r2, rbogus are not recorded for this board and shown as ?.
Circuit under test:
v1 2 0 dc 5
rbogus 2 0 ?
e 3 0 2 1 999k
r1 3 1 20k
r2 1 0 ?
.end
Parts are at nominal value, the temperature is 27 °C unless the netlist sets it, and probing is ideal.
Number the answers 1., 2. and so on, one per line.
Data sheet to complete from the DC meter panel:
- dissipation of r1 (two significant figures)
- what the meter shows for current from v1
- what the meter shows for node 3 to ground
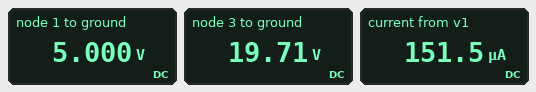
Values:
1. 11 mW
2. 151.5 µA
3. 19.71 V
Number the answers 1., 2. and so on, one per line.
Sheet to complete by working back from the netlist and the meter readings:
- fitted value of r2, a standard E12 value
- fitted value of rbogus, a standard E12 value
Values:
1. 6.8 kΩ
2. 33 kΩ
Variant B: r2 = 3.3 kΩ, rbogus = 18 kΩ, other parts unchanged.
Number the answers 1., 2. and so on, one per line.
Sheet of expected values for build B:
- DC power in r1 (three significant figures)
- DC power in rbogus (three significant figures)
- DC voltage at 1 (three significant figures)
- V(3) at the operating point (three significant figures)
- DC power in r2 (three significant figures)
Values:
1. 45.9 mW
2. 1.39 mW
3. 5.00 V
4. 35.3 V
5. 7.58 mW
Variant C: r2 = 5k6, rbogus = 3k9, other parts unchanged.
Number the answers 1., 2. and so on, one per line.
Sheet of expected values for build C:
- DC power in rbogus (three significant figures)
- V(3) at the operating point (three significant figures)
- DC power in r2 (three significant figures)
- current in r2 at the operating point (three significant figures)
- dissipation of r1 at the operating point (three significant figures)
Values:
1. 6.41 mW
2. 22.9 V
3. 4.46 mW
4. 893 µA
5. 15.9 mW
